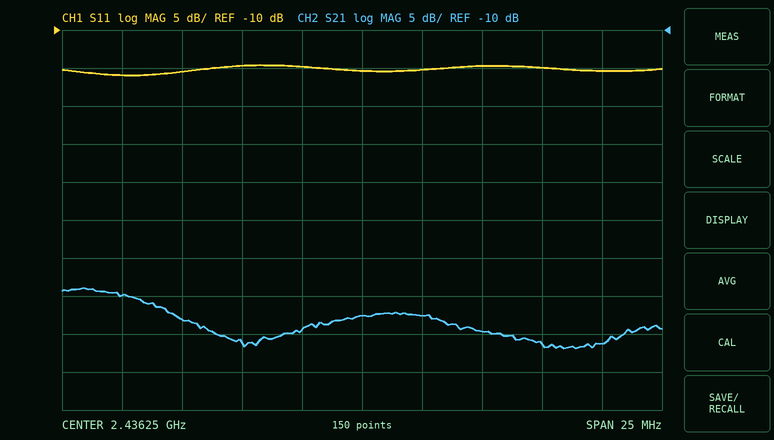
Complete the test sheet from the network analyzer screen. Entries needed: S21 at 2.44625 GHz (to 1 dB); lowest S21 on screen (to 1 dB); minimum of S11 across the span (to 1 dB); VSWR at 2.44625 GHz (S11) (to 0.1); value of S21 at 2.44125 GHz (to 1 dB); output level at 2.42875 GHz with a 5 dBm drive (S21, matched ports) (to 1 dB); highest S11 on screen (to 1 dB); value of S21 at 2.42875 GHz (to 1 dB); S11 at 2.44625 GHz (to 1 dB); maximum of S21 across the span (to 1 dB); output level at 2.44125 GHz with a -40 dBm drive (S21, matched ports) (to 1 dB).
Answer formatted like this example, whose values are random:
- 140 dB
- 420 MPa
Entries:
- -51 dB
- -52 dB
- -16 dB
- 1.4
- -50 dB
- -43 dBm
- -15 dB
- -48 dB
- -15 dB
- -44 dB
- -90 dBm
